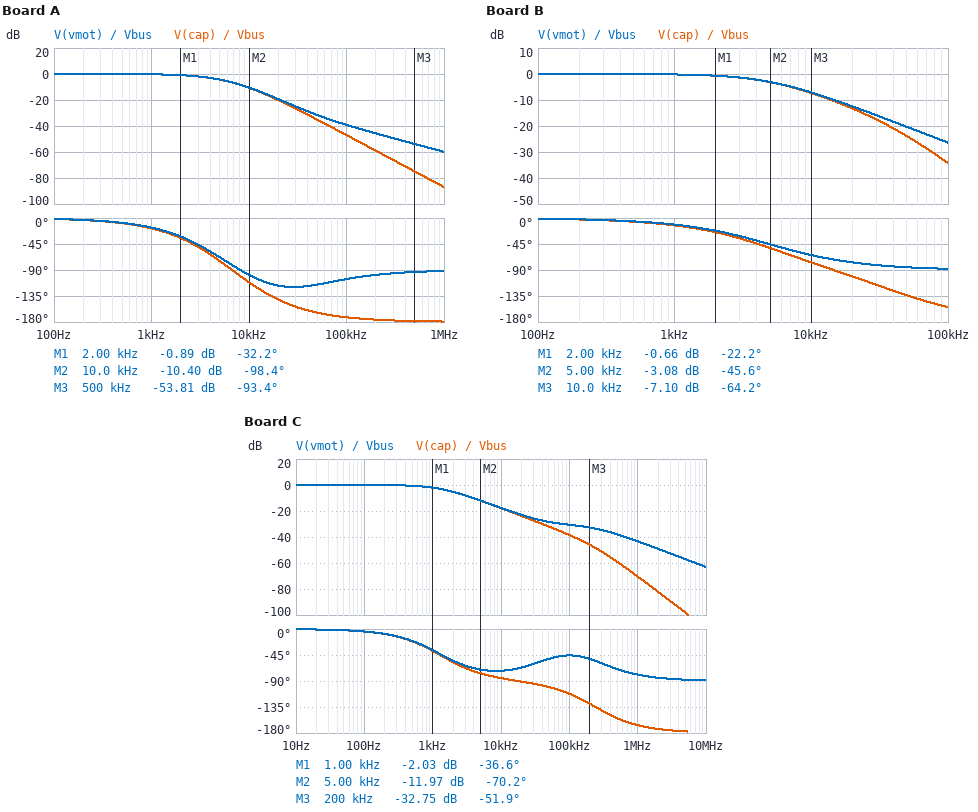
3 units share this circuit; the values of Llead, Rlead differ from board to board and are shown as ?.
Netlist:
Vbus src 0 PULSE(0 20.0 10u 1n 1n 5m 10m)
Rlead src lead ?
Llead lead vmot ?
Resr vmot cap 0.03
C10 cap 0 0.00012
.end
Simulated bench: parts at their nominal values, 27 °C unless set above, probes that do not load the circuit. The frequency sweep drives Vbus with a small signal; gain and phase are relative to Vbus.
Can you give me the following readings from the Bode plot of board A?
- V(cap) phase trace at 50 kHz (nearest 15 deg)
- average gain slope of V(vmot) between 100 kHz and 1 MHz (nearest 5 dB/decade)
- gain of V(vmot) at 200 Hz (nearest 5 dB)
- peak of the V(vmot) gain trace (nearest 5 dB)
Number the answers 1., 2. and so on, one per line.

1. -165 deg
2. -20 dB/decade
3. 0 dB
4. 0 dB
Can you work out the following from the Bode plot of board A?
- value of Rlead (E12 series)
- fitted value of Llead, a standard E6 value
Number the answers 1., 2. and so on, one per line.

1. 0.39 Ω
2. 4.7 µH
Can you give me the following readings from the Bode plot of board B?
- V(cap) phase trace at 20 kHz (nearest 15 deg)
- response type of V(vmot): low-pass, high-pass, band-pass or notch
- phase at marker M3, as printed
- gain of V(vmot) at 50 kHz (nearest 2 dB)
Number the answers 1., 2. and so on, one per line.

1. -105 deg
2. low-pass
3. -64.2 deg
4. -20 dB
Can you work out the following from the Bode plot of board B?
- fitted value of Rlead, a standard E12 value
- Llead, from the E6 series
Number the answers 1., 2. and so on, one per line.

1. 0.27 Ω
2. 1 µH
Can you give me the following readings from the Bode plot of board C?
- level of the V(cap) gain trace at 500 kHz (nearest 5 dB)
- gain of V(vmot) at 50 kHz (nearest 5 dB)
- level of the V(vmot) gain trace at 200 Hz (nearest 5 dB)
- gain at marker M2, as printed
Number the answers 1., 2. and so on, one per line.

1. -60 dB
2. -30 dB
3. 0 dB
4. -11.97 dB
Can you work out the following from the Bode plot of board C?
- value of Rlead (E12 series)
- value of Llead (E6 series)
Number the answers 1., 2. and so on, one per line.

1. 1 Ω
2. 680 nH
